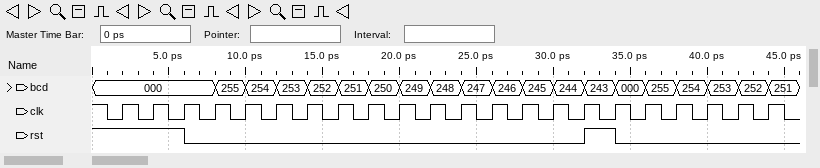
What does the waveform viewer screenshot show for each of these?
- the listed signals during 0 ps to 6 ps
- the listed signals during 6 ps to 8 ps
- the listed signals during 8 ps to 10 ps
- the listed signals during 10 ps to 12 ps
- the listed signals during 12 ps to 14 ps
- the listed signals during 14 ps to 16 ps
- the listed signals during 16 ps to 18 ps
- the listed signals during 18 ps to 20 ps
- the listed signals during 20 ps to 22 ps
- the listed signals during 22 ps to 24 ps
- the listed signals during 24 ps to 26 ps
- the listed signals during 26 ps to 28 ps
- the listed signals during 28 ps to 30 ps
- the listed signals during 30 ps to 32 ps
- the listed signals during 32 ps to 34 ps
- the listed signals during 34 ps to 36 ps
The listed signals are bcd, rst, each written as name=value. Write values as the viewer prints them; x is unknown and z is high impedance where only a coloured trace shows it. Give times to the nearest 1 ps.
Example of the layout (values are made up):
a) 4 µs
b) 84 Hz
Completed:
a) bcd=000, rst=1
b) bcd=000, rst=0
c) bcd=255, rst=0
d) bcd=254, rst=0
e) bcd=253, rst=0
f) bcd=252, rst=0
g) bcd=251, rst=0
h) bcd=250, rst=0
i) bcd=249, rst=0
j) bcd=248, rst=0
k) bcd=247, rst=0
l) bcd=246, rst=0
m) bcd=245, rst=0
n) bcd=244, rst=0
o) bcd=243, rst=1
p) bcd=000, rst=0
